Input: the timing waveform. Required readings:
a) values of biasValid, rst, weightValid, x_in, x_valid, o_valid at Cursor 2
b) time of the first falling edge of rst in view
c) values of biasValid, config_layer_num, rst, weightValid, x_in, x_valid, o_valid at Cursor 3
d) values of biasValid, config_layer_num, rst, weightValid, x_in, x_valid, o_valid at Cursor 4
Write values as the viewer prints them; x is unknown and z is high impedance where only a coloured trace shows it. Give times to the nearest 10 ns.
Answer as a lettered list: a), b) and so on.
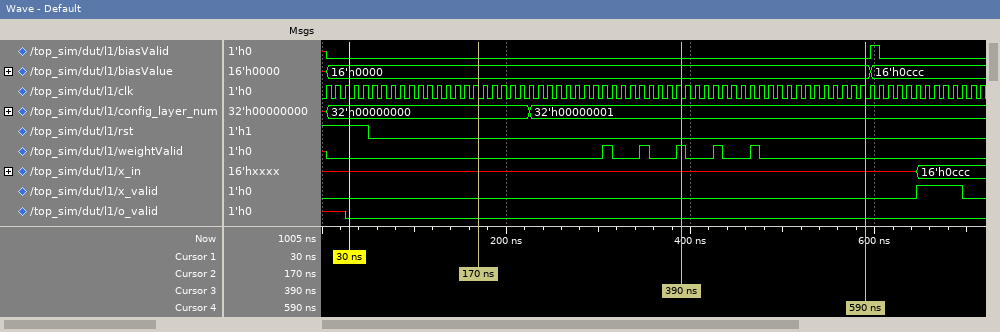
a) biasValid=0, rst=0, weightValid=0, x_in=x, x_valid=0, o_valid=0
b) 50 ns
c) biasValid=0, config_layer_num=32'h00000001, rst=0, weightValid=1, x_in=x, x_valid=0, o_valid=0
d) biasValid=0, config_layer_num=32'h00000001, rst=0, weightValid=0, x_in=x, x_valid=0, o_valid=0
